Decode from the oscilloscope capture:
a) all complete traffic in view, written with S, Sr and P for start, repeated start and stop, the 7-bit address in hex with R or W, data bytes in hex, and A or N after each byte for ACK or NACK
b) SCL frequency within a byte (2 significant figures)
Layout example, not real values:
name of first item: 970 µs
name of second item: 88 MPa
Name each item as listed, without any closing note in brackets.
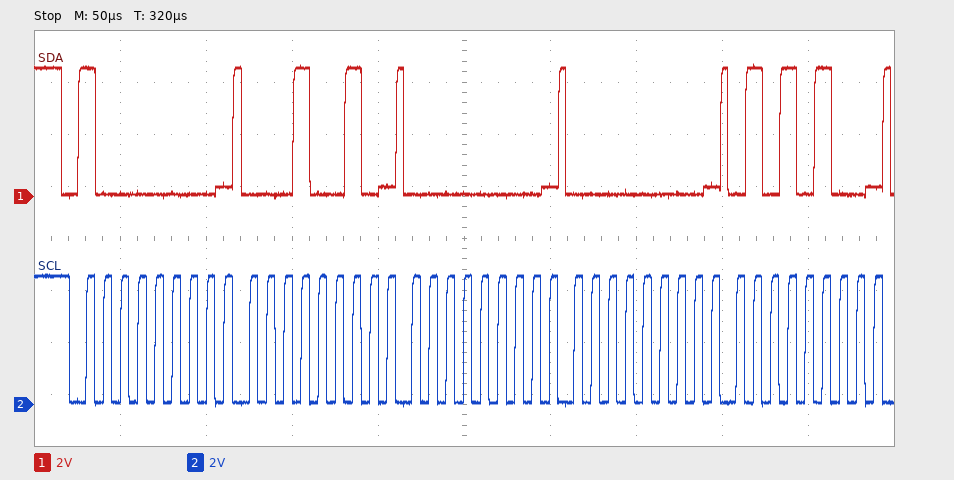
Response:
all complete traffic in view, written with S, Sr and P for start, repeated start and stop, the 7-bit address in hex with R or W, data bytes in hex, and A or N after each byte for ACK or NACK: S 40W A 12 A 00 A 00 A 54 A
SCL frequency within a byte: 100 kHz
